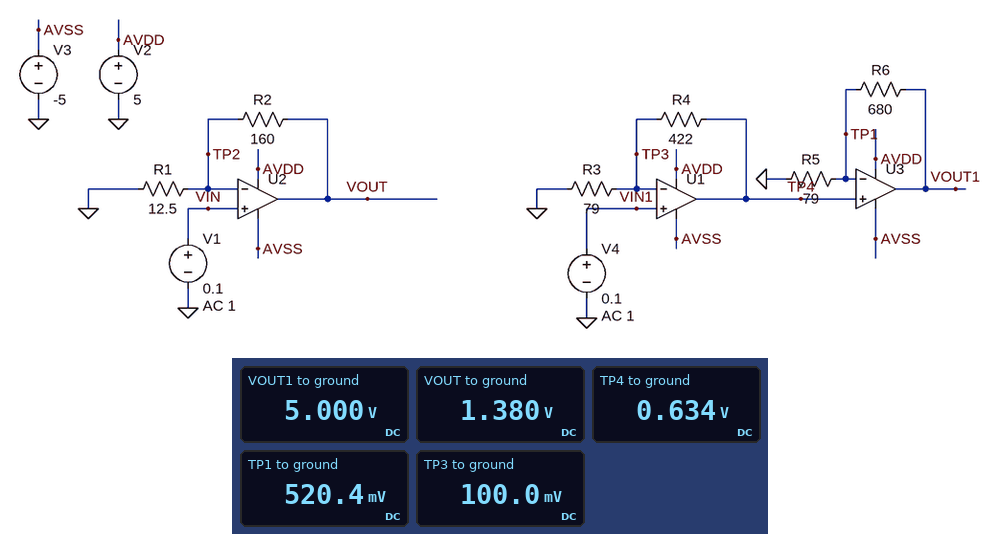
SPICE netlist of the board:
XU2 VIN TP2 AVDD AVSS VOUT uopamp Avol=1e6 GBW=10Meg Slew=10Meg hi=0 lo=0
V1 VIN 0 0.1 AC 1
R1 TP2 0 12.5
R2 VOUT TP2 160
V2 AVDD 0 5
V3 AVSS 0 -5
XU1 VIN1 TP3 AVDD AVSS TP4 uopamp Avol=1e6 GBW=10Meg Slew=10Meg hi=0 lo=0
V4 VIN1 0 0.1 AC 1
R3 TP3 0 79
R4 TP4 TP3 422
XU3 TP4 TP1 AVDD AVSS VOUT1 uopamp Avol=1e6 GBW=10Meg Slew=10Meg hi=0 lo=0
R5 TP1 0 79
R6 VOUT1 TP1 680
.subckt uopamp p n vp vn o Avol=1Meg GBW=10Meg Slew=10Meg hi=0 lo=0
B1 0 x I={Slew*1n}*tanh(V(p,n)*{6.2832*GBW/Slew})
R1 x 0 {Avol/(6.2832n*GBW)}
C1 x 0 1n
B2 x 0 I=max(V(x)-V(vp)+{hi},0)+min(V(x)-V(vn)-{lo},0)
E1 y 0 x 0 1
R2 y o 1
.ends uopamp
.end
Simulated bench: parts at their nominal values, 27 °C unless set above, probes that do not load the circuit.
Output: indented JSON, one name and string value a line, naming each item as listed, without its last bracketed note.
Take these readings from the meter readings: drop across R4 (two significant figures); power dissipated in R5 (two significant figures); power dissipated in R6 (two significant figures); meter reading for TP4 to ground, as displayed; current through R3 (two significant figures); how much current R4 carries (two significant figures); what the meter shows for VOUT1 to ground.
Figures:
{
  "drop across R4": "530 mV",
  "power dissipated in R5": "3.4 mW",
  "power dissipated in R6": "30 mW",
  "meter reading for TP4 to ground, as displayed": "0.634 V",
  "current through R3": "1.3 mA",
  "how much current R4 carries": "1.3 mA",
  "what the meter shows for VOUT1 to ground": "5.000 V"
}
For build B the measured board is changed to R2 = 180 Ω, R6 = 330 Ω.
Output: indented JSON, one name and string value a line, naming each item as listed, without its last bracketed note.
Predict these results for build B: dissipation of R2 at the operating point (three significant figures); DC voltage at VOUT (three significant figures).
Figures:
{
  "dissipation of R2 at the operating point": "11.5 mW",
  "DC voltage at VOUT": "1.54 V"
}
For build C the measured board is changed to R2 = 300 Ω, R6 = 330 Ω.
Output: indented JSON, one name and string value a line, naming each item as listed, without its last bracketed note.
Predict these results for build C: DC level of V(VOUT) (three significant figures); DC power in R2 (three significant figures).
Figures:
{
  "DC level of V(VOUT)": "2.50 V",
  "DC power in R2": "19.2 mW"
}
